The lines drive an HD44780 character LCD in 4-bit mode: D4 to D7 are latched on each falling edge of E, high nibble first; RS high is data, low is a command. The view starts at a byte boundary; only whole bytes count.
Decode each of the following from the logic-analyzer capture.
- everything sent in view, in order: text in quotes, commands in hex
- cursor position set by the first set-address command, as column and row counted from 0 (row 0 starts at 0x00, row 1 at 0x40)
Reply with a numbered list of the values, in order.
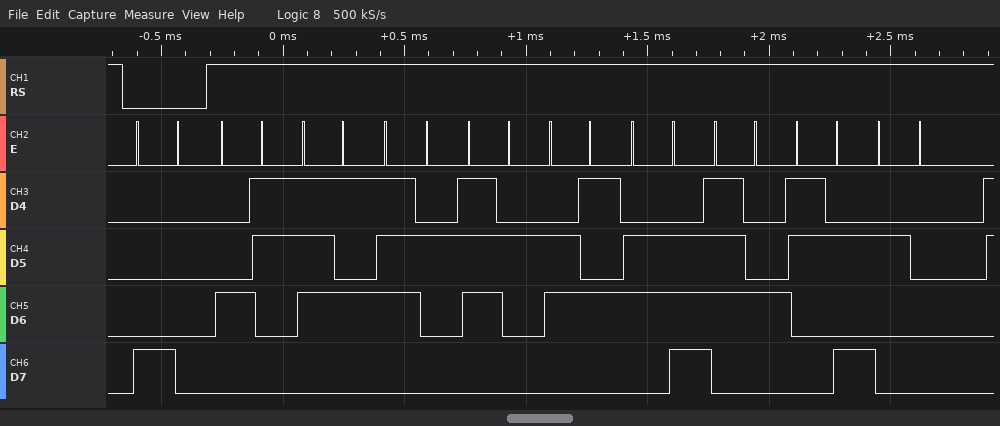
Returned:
1. 0x80 "Current: "
2. column 0, row 0
